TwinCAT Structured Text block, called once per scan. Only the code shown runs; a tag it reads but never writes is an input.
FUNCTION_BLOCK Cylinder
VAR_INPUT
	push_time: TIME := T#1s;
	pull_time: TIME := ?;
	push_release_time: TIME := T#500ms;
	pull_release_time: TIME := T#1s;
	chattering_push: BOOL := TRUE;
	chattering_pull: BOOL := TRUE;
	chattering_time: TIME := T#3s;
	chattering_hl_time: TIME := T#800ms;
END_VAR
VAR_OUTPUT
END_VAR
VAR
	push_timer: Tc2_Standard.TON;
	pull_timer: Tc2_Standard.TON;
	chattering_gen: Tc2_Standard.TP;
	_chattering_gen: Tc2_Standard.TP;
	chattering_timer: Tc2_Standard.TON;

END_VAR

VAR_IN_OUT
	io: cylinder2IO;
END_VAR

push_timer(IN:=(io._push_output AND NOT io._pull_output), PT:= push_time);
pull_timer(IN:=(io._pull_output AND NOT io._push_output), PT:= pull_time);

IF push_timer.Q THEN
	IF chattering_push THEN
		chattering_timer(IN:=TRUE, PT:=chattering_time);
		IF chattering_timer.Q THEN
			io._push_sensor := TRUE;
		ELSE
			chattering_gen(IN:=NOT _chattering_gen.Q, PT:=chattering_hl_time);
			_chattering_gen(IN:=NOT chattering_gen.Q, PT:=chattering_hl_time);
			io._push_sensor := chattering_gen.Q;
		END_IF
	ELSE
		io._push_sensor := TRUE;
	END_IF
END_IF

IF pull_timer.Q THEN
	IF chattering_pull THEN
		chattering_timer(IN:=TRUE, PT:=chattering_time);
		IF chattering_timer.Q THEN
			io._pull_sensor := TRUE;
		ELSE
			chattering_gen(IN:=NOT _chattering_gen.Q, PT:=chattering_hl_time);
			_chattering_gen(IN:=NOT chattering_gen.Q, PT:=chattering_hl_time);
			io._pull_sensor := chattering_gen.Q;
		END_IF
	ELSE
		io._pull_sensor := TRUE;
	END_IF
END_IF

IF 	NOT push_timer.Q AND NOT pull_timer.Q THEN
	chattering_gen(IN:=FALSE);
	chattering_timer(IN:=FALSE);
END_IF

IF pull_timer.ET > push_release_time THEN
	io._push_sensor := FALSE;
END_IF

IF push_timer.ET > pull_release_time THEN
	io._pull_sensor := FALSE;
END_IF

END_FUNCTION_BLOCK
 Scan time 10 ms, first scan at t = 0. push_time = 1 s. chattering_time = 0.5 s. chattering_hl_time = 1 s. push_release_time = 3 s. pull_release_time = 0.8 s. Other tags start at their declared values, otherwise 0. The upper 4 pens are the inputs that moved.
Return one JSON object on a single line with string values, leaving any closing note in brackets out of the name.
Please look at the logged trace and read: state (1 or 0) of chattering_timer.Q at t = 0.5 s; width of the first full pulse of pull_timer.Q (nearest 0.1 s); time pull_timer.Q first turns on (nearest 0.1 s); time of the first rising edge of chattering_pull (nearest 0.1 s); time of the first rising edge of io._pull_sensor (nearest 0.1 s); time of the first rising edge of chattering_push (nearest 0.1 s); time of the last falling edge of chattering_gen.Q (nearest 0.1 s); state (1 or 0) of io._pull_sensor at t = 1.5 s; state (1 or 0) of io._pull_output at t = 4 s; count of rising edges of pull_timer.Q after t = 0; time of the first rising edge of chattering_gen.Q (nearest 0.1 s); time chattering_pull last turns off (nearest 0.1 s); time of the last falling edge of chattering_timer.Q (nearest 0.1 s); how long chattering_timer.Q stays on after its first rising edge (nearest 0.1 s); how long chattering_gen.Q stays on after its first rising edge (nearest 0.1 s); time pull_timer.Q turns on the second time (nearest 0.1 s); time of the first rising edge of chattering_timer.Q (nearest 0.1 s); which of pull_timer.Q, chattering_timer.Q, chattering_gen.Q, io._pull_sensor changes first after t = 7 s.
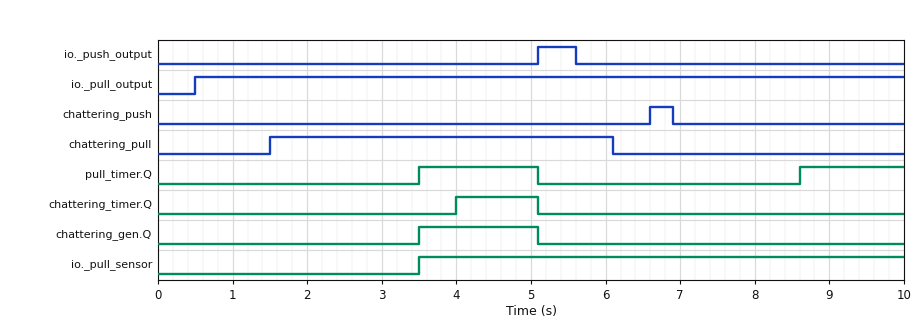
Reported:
{"state (1 or 0) of chattering_timer.Q at t = 0.5 s": "0", "width of the first full pulse of pull_timer.Q": "1.6 s", "time pull_timer.Q first turns on": "3.5 s", "time of the first rising edge of chattering_pull": "1.5 s", "time of the first rising edge of io._pull_sensor": "3.5 s", "time of the first rising edge of chattering_push": "6.6 s", "time of the last falling edge of chattering_gen.Q": "5.1 s", "state (1 or 0) of io._pull_sensor at t = 1.5 s": "0", "state (1 or 0) of io._pull_output at t = 4 s": "1", "count of rising edges of pull_timer.Q after t = 0": "2", "time of the first rising edge of chattering_gen.Q": "3.5 s", "time chattering_pull last turns off": "6.1 s", "time of the last falling edge of chattering_timer.Q": "5.1 s", "how long chattering_timer.Q stays on after its first rising edge": "1.1 s", "how long chattering_gen.Q stays on after its first rising edge": "1.6 s", "time pull_timer.Q turns on the second time": "8.6 s", "time of the first rising edge of chattering_timer.Q": "4.0 s", "which of pull_timer.Q, chattering_timer.Q, chattering_gen.Q, io._pull_sensor changes first after t = 7 s": "pull_timer.Q"}
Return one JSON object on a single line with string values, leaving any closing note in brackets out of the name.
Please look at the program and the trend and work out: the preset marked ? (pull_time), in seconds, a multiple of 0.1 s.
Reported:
{"the preset marked ? (pull_time), in seconds, a multiple of 0.1 s": "3.0 s"}
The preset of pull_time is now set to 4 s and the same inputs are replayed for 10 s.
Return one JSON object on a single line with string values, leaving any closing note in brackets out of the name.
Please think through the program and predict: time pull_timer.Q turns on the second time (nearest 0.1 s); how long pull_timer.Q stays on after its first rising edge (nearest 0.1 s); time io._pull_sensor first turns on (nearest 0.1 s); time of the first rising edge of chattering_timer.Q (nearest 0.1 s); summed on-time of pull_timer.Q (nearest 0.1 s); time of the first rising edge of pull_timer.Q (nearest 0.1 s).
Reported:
{"time pull_timer.Q turns on the second time": "9.6 s", "how long pull_timer.Q stays on after its first rising edge": "0.6 s", "time io._pull_sensor first turns on": "4.5 s", "time of the first rising edge of chattering_timer.Q": "5.0 s", "summed on-time of pull_timer.Q": "1.0 s", "time of the first rising edge of pull_timer.Q": "4.5 s"}
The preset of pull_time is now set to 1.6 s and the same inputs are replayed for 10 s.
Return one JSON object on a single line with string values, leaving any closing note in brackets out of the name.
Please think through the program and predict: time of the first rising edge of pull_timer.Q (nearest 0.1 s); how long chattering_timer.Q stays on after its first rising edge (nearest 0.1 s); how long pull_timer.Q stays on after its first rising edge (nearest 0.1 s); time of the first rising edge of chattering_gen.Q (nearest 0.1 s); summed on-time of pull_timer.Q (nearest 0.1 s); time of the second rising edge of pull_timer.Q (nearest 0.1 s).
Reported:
{"time of the first rising edge of pull_timer.Q": "2.1 s", "how long chattering_timer.Q stays on after its first rising edge": "2.5 s", "how long pull_timer.Q stays on after its first rising edge": "3.0 s", "time of the first rising edge of chattering_gen.Q": "2.1 s", "summed on-time of pull_timer.Q": "5.8 s", "time of the second rising edge of pull_timer.Q": "7.2 s"}
